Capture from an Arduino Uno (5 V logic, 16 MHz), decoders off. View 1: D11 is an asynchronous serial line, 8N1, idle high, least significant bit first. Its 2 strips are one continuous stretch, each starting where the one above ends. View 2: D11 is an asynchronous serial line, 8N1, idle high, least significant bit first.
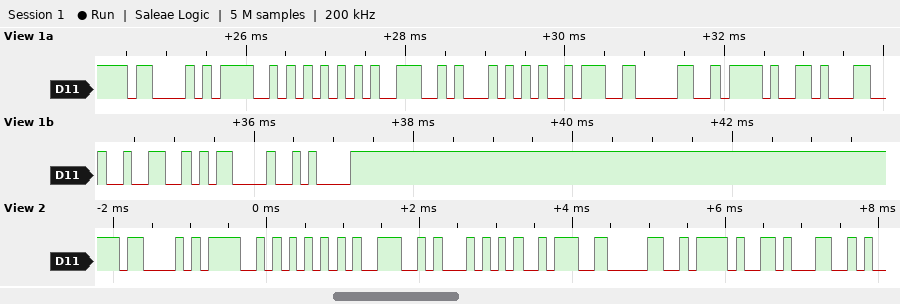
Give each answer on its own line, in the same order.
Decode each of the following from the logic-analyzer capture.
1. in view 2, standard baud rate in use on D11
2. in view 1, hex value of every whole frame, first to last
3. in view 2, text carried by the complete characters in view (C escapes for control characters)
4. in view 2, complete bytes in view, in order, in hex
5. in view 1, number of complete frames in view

9600 baud
43 4F 55 4E 54 3A 30 2F 31 32 0D 0A
"COUNT:0/1"
0x43 0x4F 0x55 0x4E 0x54 0x3A 0x30 0x2F 0x31
12
